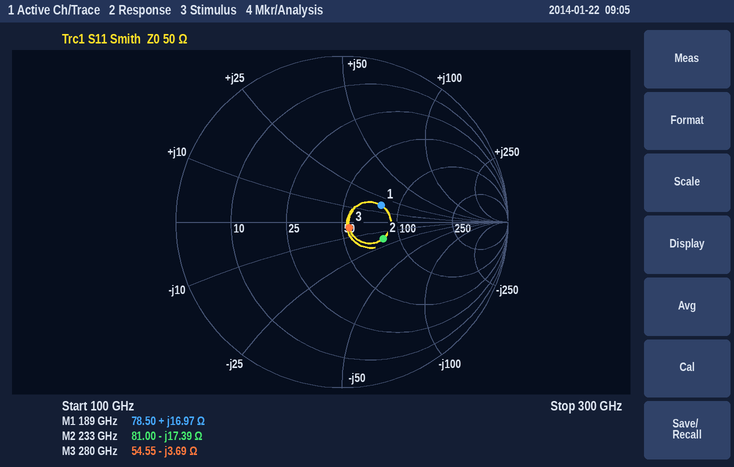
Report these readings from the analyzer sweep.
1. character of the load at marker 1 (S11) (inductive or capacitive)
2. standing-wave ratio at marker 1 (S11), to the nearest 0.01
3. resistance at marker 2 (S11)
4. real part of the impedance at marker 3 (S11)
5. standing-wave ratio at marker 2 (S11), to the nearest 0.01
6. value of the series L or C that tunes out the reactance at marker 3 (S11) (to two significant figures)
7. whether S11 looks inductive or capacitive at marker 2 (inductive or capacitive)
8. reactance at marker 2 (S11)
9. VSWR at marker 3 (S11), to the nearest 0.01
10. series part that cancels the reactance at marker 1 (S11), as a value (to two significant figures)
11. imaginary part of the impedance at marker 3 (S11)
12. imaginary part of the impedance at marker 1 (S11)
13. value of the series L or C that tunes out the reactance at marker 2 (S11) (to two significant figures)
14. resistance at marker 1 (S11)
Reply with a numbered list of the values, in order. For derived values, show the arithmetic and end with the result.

1. inductive
2. 1.69
3. 81.00 Ω
4. 54.55 Ω
5. 1.74
6. L = 3.69 Ω/(2π × 280 GHz) ≈ 2.1 pH
7. capacitive
8. -17.39 Ω
9. 1.12
10. C = 1/(2π × 189 GHz × 16.97 Ω) ≈ 50 fF
11. -3.69 Ω
12. +16.97 Ω
13. L = 17.39 Ω/(2π × 233 GHz) ≈ 12 pH
14. 78.50 Ω
